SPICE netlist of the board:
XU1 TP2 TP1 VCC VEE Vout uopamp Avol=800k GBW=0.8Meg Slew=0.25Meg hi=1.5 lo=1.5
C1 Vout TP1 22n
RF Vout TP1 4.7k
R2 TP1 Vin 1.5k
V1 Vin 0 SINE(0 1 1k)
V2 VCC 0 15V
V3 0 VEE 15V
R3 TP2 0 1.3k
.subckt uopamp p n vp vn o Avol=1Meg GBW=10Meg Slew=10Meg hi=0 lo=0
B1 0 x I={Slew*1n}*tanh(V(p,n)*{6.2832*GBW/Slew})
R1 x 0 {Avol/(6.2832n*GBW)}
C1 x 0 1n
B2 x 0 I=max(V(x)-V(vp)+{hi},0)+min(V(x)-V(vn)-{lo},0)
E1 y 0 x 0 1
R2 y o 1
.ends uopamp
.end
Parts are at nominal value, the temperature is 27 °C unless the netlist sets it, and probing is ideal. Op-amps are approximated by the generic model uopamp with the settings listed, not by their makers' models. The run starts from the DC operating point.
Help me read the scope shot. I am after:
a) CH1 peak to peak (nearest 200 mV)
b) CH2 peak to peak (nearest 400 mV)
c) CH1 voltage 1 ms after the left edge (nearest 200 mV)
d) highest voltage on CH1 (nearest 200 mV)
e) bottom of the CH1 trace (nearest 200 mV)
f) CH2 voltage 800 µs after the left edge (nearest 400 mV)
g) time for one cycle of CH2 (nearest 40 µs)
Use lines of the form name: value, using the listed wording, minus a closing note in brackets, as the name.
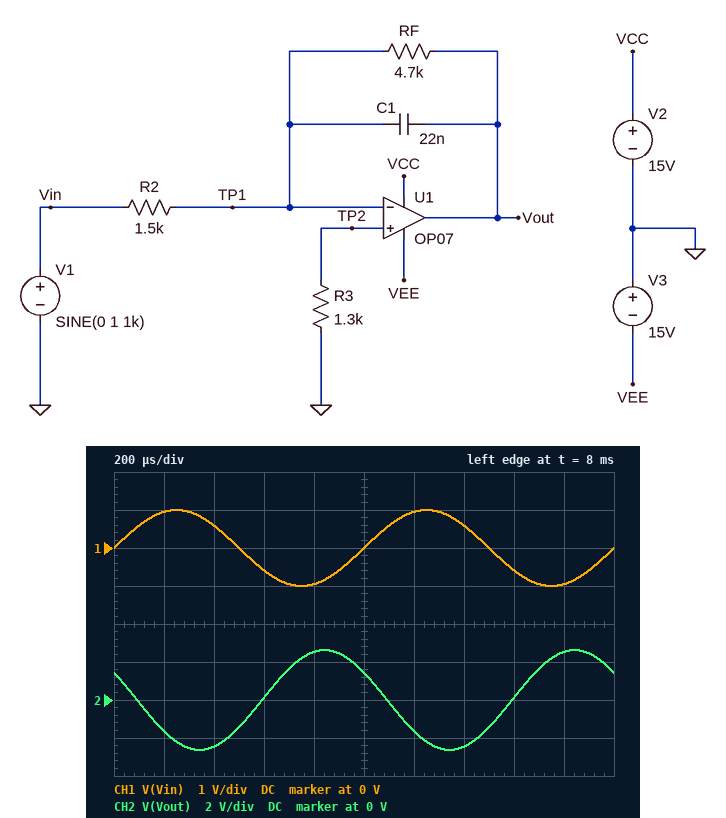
CH1 peak to peak: 2.0 V
CH2 peak to peak: 5.2 V
CH1 voltage 1 ms after the left edge: 0 V
highest voltage on CH1: 1.0 V
bottom of the CH1 trace: -1.0 V
CH2 voltage 800 µs after the left edge: 2.4 V
time for one cycle of CH2: 1.00 ms
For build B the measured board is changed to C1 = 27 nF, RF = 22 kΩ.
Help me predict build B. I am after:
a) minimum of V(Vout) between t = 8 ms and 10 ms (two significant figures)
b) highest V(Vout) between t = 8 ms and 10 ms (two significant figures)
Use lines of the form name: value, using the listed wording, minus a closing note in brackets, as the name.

minimum of V(Vout) between t = 8 ms and 10 ms: -3.8 V
highest V(Vout) between t = 8 ms and 10 ms: 3.8 V
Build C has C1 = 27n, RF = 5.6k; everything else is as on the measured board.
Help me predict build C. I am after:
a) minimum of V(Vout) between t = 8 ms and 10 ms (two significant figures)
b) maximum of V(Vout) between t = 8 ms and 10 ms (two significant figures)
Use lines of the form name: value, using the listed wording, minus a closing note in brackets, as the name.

minimum of V(Vout) between t = 8 ms and 10 ms: -2.7 V
maximum of V(Vout) between t = 8 ms and 10 ms: 2.7 V
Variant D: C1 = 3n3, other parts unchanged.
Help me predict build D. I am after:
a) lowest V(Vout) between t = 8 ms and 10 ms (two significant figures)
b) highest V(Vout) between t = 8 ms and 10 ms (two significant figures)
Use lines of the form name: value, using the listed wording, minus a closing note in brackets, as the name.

lowest V(Vout) between t = 8 ms and 10 ms: -3.1 V
highest V(Vout) between t = 8 ms and 10 ms: 3.1 V
